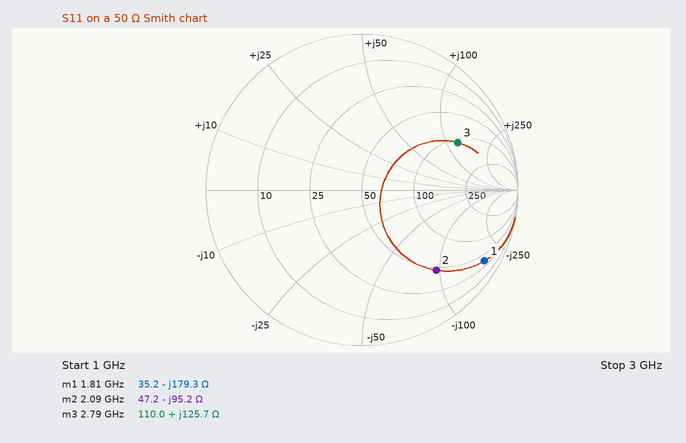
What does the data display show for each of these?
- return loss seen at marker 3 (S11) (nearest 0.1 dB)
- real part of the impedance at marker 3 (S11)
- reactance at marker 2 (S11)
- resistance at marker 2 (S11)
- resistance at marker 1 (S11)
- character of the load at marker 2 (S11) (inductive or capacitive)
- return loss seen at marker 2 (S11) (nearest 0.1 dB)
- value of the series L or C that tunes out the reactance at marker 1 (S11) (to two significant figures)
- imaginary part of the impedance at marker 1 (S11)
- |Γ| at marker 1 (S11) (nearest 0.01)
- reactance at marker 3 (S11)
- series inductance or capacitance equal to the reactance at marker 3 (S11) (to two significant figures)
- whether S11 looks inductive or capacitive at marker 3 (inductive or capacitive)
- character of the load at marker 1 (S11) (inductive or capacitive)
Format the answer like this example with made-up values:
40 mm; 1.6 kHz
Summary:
3.3 dB; 110.0 Ω; -95.2 Ω; 47.2 Ω; 35.2 Ω; capacitive; 3.1 dB; 16 nH; -179.3 Ω; 0.91; +125.7 Ω; 7.2 nH; inductive; capacitive
